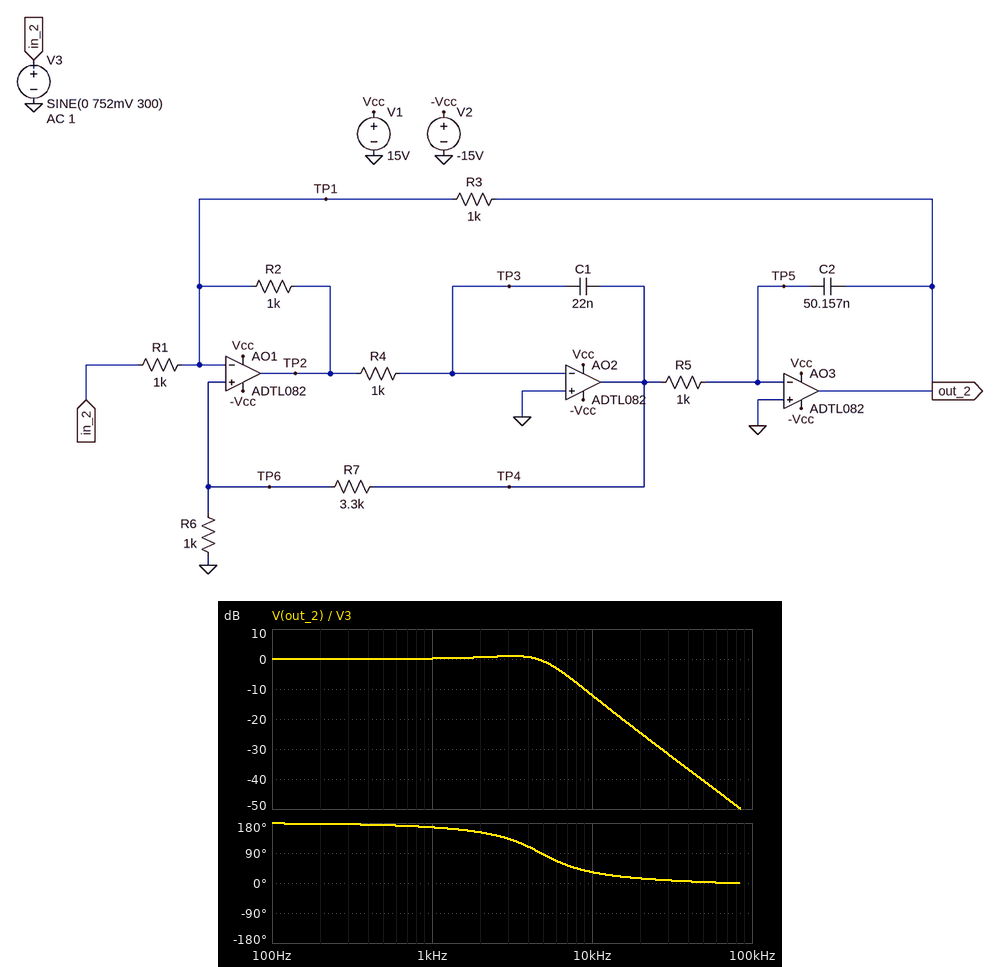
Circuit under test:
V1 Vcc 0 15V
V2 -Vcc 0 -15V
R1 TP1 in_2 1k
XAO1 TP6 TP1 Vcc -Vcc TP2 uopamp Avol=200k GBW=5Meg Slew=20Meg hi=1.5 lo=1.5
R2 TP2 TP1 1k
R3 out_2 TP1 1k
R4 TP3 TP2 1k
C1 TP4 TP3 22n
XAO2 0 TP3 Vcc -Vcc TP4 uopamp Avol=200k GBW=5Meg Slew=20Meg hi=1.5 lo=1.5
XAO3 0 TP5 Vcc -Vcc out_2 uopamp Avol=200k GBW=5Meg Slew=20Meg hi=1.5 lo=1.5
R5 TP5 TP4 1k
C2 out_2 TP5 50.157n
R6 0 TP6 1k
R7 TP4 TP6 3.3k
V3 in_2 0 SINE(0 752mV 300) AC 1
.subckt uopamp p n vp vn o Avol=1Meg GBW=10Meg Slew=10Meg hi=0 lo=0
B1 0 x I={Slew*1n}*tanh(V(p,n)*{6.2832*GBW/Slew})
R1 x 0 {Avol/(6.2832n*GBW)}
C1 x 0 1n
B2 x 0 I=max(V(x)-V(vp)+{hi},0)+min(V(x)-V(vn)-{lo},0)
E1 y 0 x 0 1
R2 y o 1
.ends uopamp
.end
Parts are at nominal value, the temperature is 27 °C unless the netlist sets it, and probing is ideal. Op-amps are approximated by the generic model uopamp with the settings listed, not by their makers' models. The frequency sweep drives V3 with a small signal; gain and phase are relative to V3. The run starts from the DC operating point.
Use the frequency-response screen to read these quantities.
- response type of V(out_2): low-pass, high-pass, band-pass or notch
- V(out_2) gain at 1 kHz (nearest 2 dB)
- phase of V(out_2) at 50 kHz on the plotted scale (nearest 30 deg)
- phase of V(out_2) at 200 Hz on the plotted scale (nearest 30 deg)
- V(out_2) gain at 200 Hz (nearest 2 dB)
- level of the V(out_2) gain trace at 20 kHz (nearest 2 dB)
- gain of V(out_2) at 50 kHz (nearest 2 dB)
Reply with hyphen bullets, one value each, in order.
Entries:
- low-pass
- 0 dB
- 0 deg
- 180 deg
- 0 dB
- -24 dB
- -40 dB
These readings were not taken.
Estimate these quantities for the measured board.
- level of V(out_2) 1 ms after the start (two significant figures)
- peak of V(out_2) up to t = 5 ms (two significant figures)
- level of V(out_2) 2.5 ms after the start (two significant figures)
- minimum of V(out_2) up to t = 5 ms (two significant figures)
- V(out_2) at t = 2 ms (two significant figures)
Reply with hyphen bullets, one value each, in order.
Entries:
- -730 mV
- 750 mV
- 750 mV
- -750 mV
- 400 mV
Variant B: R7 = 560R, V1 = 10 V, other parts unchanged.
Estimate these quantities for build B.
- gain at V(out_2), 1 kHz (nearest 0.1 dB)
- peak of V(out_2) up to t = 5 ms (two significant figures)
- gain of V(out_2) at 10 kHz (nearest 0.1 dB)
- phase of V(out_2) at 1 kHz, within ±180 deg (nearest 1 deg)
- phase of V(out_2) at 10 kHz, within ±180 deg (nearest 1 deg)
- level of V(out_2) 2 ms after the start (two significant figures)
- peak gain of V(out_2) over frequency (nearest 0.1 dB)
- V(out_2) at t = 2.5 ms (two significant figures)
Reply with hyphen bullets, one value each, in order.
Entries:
- -1.1 dB
- 740 mV
- -16.8 dB
- 148 deg
- 61 deg
- 320 mV
- 0 dB
- 730 mV
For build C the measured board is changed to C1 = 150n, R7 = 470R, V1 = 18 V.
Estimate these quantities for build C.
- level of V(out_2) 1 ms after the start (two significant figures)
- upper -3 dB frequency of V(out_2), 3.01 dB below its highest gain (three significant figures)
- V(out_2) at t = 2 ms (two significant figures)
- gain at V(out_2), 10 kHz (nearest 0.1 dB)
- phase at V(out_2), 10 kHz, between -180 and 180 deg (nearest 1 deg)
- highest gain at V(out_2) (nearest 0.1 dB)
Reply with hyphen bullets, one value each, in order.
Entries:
- -750 mV
- 2.06 kHz
- 320 mV
- -29.4 dB
- 12 deg
- 0.4 dB
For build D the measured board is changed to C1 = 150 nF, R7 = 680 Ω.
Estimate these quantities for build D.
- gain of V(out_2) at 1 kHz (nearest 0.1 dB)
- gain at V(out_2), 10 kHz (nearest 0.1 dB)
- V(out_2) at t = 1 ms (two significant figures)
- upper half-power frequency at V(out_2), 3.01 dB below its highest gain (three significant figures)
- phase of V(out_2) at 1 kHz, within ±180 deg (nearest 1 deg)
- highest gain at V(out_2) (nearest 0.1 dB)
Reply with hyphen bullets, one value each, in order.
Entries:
- 0.9 dB
- -29.3 dB
- -750 mV
- 2.13 kHz
- 141 deg
- 1.1 dB
